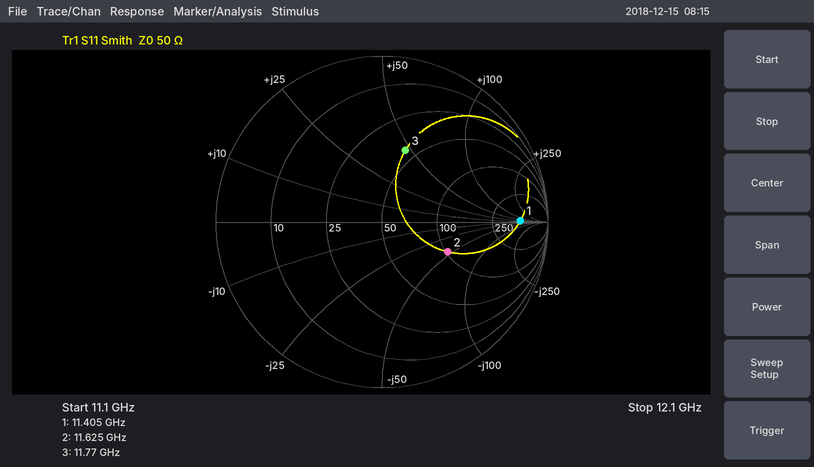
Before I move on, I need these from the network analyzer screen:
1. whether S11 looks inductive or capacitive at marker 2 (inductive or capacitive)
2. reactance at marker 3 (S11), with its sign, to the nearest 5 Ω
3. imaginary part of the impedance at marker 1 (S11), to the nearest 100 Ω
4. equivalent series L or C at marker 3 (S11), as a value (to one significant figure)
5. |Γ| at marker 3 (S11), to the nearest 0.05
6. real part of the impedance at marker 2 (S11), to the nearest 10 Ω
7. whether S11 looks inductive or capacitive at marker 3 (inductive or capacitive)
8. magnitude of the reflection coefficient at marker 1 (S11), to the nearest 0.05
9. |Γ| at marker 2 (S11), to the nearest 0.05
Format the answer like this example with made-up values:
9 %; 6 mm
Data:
capacitive; +45 Ω; 0 Ω; 600 pH; 0.45; 100 Ω; inductive; 0.85; 0.45
